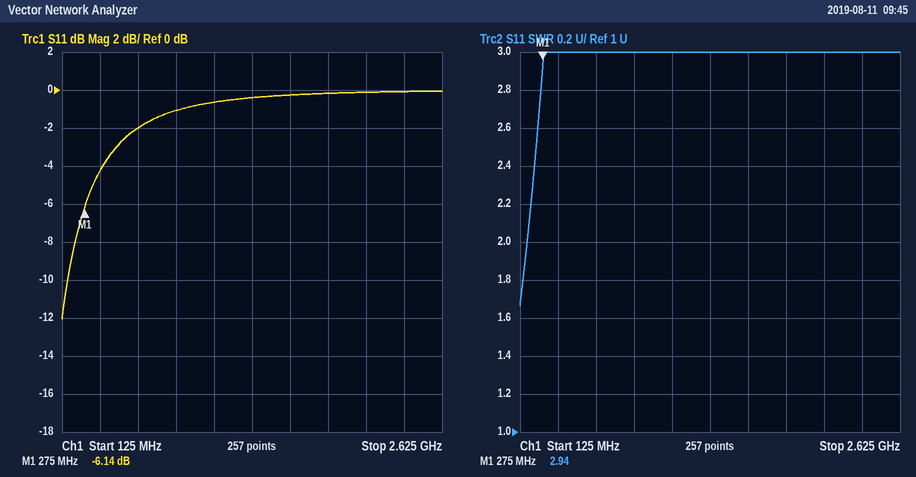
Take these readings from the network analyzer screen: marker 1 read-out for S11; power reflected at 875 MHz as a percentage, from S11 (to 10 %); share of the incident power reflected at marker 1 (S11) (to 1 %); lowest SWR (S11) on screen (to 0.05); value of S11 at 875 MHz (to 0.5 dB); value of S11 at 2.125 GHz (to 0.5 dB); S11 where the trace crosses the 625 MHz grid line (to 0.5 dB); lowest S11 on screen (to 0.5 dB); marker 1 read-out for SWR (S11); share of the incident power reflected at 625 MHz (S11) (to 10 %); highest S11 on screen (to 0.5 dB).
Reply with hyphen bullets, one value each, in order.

- -6.14 dB
- 80 %
- 24 %
- 1.65
- -1.0 dB
- 0.0 dB
- -2.0 dB
- -12.0 dB
- 2.94
- 60 %
- 0.0 dB
